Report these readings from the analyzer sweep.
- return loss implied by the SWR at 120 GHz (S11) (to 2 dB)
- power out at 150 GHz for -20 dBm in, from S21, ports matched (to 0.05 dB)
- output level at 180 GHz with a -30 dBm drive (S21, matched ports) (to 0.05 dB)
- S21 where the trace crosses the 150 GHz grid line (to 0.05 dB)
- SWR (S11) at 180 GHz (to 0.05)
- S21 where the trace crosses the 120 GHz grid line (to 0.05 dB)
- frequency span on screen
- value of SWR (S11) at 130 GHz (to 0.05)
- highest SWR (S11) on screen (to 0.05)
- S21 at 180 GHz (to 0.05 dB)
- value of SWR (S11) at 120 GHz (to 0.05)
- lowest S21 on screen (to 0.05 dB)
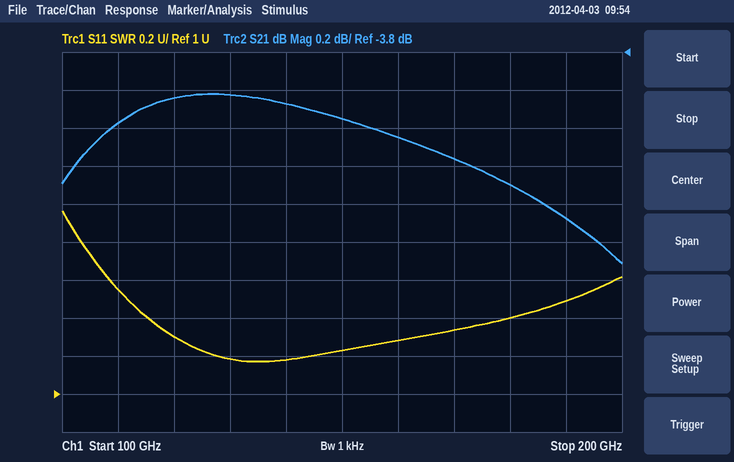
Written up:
18 dB
-24.15 dBm
-34.50 dBm
-4.15 dB
1.40
-4.05 dB
100 GHz
1.20
1.95
-4.50 dB
1.30
-4.90 dB
